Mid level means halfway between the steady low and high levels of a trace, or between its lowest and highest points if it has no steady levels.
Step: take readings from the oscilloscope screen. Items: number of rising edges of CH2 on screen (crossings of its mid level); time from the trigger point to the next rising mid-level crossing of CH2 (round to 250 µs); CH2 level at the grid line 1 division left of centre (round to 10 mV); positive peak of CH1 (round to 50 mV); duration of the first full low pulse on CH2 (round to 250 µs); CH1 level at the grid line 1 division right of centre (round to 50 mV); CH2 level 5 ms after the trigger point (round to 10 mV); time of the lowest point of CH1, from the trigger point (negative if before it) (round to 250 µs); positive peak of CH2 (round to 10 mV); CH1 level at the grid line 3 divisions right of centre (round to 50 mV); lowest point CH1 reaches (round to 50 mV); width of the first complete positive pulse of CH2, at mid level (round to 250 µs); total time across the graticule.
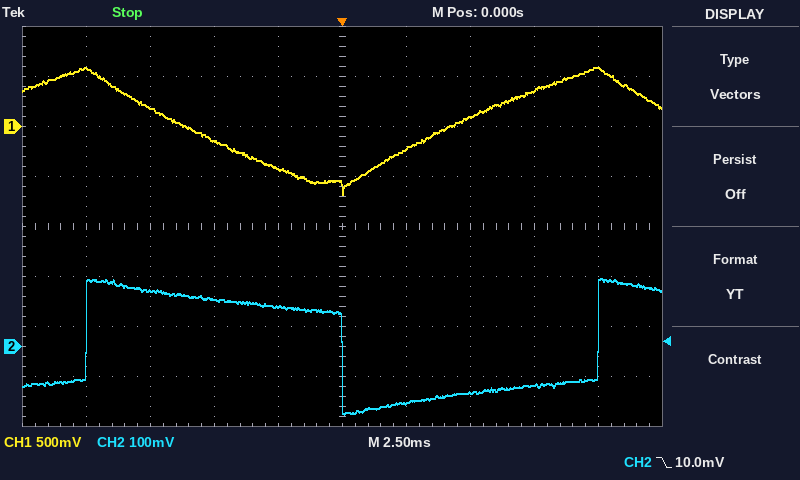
2
10.00 ms
80 mV
600 mV
10.00 ms
-200 mV
-90 mV
0.00 ms
140 mV
350 mV
-700 mV
10.00 ms
25 ms
